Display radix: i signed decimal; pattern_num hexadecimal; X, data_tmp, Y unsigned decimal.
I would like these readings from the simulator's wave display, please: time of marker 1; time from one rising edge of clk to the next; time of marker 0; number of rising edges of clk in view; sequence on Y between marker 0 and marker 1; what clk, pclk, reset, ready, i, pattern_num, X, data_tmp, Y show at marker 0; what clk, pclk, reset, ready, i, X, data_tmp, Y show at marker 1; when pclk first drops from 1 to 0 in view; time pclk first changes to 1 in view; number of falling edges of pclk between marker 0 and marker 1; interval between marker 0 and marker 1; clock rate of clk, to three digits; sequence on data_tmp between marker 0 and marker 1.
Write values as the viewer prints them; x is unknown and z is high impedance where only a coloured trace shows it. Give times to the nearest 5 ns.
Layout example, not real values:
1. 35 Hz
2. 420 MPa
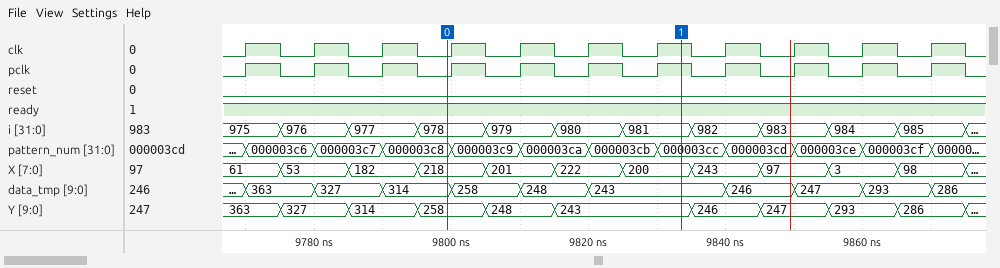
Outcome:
1. 9835 ns
2. 10 ns
3. 9800 ns
4. 11
5. 258, 248, 243
6. clk=0, pclk=0, reset=0, ready=1, i=978, pattern_num=000003c8, X=218, data_tmp=314, Y=258
7. clk=1, pclk=1, reset=0, ready=1, i=981, X=200, data_tmp=243, Y=243
8. 9775 ns
9. 9770 ns
10. 3
11. 35 ns
12. 100 MHz
13. 314, 258, 248, 243
